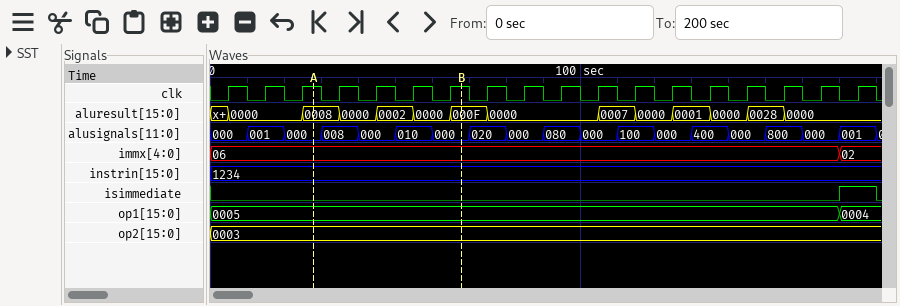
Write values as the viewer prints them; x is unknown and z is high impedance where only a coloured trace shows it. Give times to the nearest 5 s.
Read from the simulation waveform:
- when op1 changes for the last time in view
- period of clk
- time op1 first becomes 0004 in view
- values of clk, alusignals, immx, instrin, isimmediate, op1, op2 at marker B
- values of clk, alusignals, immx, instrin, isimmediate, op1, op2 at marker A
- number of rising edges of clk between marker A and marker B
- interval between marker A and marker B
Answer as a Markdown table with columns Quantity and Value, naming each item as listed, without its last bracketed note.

| Quantity | Value |
|---|---|
| when op1 changes for the last time in view | 170 s |
| period of clk | 10 s |
| time op1 first becomes 0004 in view | 170 s |
| values of clk, alusignals, immx, instrin, isimmediate, op1, op2 at marker B | clk=1, alusignals=000, immx=06, instrin=1234, isimmediate=0, op1=0005, op2=0003 |
| values of clk, alusignals, immx, instrin, isimmediate, op1, op2 at marker A | clk=1, alusignals=000, immx=06, instrin=1234, isimmediate=0, op1=0005, op2=0003 |
| number of rising edges of clk between marker A and marker B | 4 |
| interval between marker A and marker B | 40 s |
